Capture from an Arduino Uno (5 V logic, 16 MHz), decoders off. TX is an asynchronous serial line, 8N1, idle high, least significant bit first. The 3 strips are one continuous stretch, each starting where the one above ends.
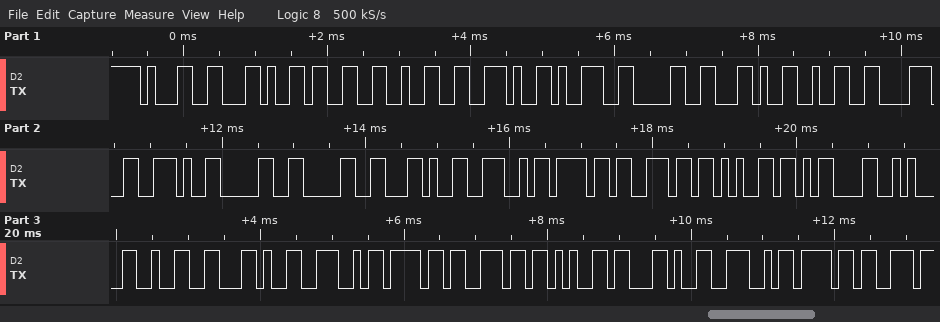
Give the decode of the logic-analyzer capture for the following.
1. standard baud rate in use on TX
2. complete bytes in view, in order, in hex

9600 baud
31 2C 33 32 2E 39 30 2C 32 38 2E 30 30 2C 4E 6F 6E 65 0D 0A 32 2C 4E 6F 6E 65 2C 4E 6F
